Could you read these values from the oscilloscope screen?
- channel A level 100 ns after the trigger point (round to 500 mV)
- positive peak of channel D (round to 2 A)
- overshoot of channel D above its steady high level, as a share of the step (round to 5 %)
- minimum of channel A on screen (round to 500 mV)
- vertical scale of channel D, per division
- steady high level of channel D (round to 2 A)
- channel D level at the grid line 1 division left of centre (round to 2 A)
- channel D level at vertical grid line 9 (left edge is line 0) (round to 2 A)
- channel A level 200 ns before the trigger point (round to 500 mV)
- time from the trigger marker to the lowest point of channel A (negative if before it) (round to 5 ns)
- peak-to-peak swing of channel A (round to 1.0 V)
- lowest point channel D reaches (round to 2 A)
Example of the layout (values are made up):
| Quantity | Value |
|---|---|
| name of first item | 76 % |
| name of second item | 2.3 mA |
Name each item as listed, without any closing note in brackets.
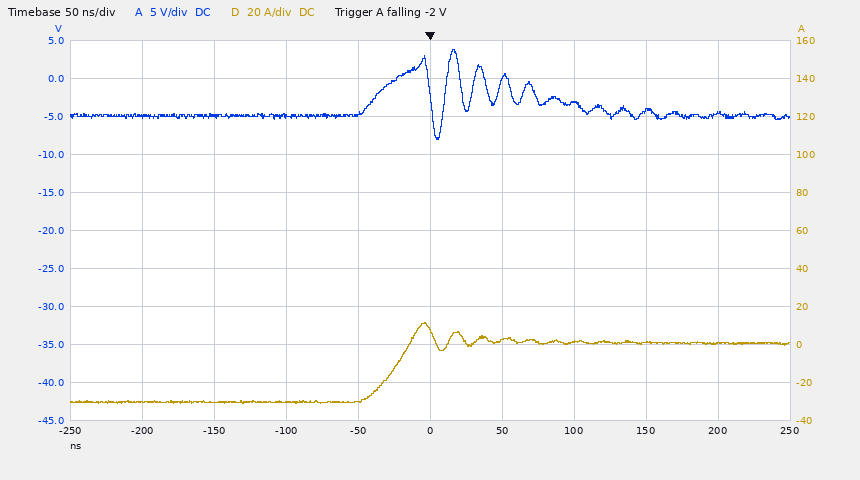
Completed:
| Quantity | Value |
|---|---|
| channel A level 100 ns after the trigger point | -3.0 V |
| positive peak of channel D | 12 A |
| overshoot of channel D above its steady high level, as a share of the step | 35 % |
| minimum of channel A on screen | -8.0 V |
| vertical scale of channel D, per division | 20 A |
| steady high level of channel D | 0 A |
| channel D level at the grid line 1 division left of centre | -30 A |
| channel D level at vertical grid line 9 (left edge is line 0) | 0 A |
| channel A level 200 ns before the trigger point | -5.0 V |
| time from the trigger marker to the lowest point of channel A (negative if before it) | +5 ns |
| peak-to-peak swing of channel A | 12.0 V |
| lowest point channel D reaches | -32 A |
